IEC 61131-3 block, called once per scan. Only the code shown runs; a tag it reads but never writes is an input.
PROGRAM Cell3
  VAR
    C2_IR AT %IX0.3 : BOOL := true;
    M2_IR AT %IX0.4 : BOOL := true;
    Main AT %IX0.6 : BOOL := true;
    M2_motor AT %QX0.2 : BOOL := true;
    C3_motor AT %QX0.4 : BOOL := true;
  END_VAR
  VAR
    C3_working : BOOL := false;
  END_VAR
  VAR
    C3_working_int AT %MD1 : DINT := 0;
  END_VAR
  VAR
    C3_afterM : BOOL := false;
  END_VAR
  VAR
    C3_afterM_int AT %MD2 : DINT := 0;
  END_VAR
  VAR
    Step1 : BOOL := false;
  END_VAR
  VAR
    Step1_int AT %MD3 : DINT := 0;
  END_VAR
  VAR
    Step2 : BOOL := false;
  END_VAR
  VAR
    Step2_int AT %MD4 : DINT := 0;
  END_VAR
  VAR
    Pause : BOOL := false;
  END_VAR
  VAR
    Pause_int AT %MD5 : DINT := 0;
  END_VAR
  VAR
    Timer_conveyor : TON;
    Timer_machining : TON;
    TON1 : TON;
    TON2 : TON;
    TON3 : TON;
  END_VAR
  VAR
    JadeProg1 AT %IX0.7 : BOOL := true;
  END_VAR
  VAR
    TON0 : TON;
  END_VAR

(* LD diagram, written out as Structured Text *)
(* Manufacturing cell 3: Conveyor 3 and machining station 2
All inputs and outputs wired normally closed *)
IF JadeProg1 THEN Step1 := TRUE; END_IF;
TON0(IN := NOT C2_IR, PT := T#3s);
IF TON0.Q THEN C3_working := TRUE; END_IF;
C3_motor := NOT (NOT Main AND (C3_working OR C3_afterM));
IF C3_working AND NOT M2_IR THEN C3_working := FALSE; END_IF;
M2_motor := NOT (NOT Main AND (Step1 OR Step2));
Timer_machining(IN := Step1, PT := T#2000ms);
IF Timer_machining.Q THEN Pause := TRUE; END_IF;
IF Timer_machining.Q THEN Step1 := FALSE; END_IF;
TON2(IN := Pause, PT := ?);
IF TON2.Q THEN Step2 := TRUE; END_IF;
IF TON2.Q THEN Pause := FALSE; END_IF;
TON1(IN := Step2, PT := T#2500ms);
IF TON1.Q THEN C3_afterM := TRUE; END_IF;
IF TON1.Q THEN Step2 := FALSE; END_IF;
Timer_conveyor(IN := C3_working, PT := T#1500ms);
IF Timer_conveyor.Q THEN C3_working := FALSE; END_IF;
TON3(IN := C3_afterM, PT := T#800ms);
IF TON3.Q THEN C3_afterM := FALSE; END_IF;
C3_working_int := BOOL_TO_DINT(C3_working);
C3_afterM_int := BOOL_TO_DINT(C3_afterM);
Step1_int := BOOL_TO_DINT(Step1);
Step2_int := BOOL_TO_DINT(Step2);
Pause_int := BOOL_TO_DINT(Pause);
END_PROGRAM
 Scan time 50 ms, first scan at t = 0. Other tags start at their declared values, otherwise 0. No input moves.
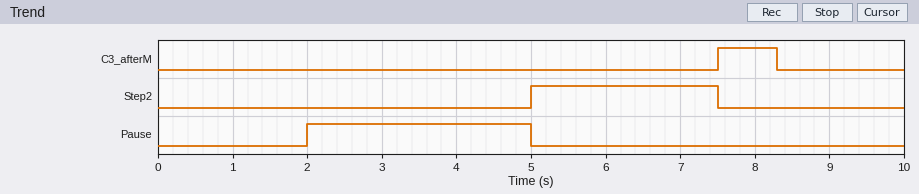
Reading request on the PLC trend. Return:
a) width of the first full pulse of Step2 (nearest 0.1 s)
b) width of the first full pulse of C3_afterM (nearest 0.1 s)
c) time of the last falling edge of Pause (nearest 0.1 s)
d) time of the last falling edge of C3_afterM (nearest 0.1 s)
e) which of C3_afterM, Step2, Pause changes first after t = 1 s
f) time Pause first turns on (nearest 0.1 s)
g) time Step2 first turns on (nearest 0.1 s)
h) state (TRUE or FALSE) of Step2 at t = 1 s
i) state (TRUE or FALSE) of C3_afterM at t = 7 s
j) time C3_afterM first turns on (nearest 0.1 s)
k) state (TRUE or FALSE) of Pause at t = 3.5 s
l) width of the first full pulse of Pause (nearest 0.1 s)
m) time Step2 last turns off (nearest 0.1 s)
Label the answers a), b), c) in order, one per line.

a) 2.5 s
b) 0.8 s
c) 5.0 s
d) 8.3 s
e) Pause
f) 2.0 s
g) 5.0 s
h) FALSE
i) FALSE
j) 7.5 s
k) TRUE
l) 3.0 s
m) 7.5 s
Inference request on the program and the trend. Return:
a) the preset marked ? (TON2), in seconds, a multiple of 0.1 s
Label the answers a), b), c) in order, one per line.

a) 3.0 s
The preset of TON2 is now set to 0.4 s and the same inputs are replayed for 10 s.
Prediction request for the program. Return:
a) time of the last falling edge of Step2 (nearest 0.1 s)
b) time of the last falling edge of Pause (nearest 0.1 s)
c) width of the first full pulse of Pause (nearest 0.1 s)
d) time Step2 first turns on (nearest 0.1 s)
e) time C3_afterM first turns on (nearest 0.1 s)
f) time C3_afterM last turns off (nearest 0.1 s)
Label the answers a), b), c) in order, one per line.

a) 4.9 s
b) 2.4 s
c) 0.4 s
d) 2.4 s
e) 4.9 s
f) 5.7 s
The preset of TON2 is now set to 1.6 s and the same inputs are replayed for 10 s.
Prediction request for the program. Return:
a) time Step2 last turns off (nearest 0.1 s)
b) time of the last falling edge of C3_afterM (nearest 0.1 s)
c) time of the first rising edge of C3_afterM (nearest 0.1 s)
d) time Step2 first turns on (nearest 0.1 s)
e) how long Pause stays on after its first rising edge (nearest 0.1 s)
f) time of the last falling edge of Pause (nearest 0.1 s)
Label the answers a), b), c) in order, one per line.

a) 6.1 s
b) 6.9 s
c) 6.1 s
d) 3.6 s
e) 1.6 s
f) 3.6 s
